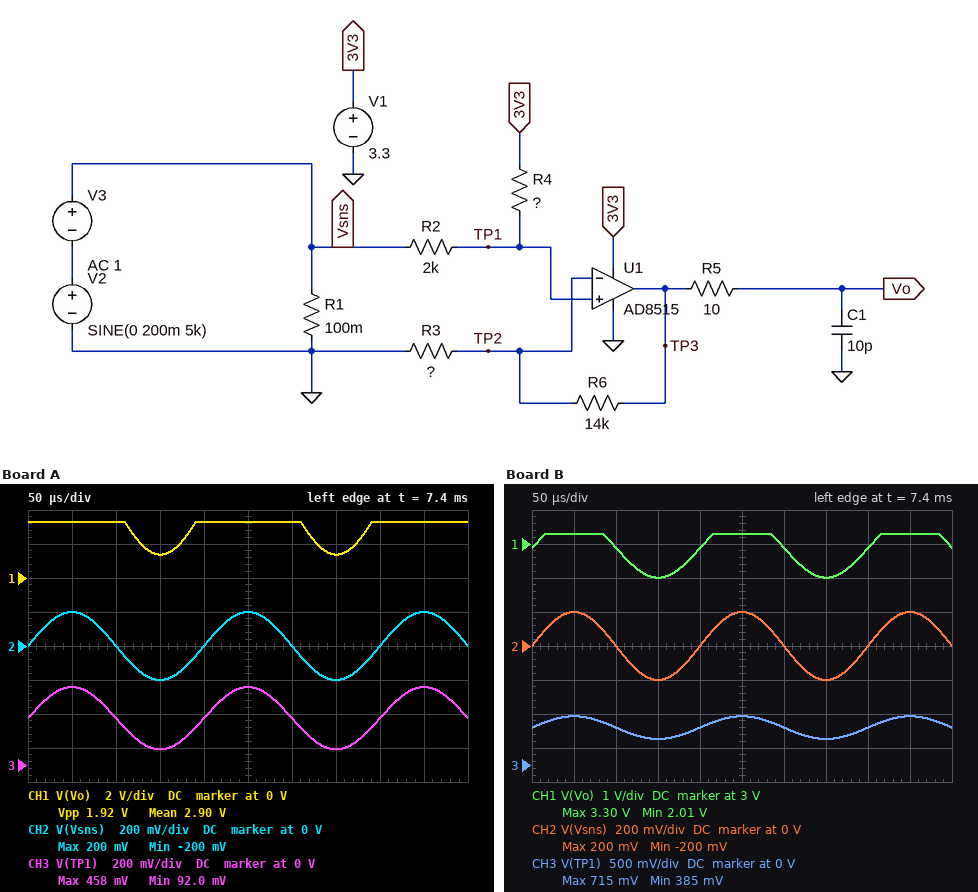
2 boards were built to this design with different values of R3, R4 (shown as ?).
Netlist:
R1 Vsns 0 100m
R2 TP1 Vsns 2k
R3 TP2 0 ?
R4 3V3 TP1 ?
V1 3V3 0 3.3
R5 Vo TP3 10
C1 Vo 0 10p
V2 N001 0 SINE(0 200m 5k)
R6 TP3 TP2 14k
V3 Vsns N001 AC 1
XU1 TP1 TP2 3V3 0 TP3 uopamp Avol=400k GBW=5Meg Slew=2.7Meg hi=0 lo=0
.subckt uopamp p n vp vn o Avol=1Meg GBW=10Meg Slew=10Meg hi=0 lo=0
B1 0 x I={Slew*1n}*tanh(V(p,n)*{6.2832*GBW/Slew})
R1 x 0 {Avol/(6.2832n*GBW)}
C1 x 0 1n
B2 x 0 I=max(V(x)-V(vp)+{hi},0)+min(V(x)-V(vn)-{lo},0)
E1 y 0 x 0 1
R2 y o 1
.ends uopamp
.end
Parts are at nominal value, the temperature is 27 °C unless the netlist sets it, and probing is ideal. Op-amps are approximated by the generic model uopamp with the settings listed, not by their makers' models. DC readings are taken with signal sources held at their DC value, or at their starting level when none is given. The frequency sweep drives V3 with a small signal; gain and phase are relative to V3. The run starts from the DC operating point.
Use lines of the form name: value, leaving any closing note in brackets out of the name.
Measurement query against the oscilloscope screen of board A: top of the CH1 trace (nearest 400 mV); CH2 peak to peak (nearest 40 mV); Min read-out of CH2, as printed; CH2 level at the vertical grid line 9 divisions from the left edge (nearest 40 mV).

top of the CH1 trace: 3.2 V
CH2 peak to peak: 400 mV
Min read-out of CH2, as printed: -200 mV
CH2 level at the vertical grid line 9 divisions from the left edge: 200 mV
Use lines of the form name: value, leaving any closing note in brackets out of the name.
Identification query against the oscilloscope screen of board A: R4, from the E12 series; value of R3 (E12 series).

R4, from the E12 series: 22 kΩ
value of R3: 1 kΩ
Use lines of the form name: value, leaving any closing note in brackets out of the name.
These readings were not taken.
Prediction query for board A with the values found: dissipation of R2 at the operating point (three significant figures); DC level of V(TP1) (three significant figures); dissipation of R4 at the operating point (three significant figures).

dissipation of R2 at the operating point: 37.8 µW
DC level of V(TP1): 275 mV
dissipation of R4 at the operating point: 416 µW
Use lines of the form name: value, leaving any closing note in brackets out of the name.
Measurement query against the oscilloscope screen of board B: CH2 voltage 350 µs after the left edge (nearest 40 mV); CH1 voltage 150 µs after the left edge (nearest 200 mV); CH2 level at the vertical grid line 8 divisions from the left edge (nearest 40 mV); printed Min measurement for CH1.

CH2 voltage 350 µs after the left edge: -200 mV
CH1 voltage 150 µs after the left edge: 2.0 V
CH2 level at the vertical grid line 8 divisions from the left edge: 0 V
printed Min measurement for CH1: 2.01 V
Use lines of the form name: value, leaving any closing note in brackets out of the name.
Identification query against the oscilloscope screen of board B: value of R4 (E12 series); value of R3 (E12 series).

value of R4: 10 kΩ
value of R3: 3.3 kΩ
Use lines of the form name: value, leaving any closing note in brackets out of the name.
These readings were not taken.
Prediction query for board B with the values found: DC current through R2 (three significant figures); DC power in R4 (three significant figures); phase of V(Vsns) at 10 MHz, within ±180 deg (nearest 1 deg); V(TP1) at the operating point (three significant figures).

DC current through R2: 275 µA
DC power in R4: 756 µW
phase of V(Vsns) at 10 MHz, within ±180 deg: 0 deg
V(TP1) at the operating point: 550 mV
